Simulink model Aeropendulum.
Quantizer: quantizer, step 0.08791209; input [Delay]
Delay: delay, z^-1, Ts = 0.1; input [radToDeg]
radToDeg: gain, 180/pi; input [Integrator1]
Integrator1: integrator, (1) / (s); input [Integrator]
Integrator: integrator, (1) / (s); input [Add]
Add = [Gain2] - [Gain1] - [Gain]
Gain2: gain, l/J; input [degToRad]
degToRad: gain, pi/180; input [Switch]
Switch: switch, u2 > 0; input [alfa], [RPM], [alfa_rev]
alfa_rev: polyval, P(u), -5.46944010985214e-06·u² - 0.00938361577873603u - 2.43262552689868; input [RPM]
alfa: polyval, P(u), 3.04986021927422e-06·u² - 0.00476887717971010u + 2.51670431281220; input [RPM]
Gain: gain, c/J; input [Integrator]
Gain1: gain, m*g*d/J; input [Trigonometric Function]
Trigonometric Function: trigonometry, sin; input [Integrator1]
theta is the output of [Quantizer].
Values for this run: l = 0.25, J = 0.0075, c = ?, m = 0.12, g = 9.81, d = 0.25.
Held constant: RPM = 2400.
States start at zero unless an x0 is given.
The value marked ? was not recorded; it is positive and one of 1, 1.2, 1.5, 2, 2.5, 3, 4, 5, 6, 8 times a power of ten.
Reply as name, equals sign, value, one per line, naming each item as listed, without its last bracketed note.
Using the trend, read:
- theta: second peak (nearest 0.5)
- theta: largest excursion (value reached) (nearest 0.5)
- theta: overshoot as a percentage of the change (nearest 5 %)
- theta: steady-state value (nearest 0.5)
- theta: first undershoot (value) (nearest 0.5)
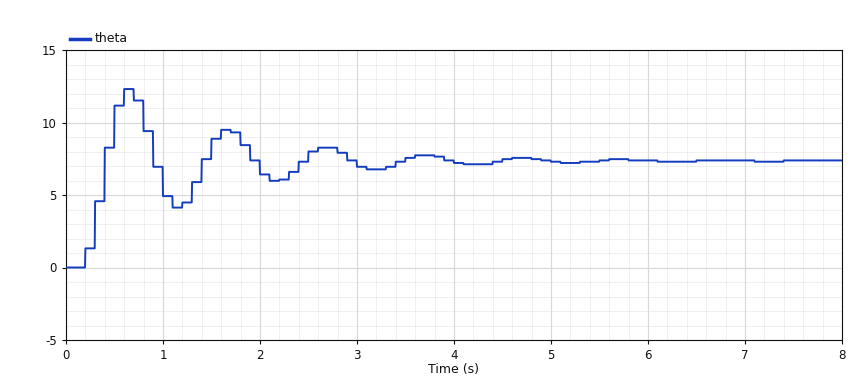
theta: second peak = 9.5
theta: largest excursion (value reached) = 12.5
theta: overshoot as a percentage of the change = 65 %
theta: steady-state value = 7.5
theta: first undershoot (value) = 4.0
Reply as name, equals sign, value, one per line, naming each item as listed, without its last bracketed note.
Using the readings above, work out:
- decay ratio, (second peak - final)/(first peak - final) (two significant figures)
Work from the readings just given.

decay ratio, (second peak - final)/(first peak - final) = 0.40
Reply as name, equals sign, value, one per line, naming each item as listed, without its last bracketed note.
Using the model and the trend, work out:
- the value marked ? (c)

the value marked ? = 0.012
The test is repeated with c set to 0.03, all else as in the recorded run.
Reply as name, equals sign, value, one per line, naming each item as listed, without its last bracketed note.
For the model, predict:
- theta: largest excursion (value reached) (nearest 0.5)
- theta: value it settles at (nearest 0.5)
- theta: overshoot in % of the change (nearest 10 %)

theta: largest excursion (value reached) = 10.0
theta: value it settles at = 7.5
theta: overshoot in % of the change = 30 %
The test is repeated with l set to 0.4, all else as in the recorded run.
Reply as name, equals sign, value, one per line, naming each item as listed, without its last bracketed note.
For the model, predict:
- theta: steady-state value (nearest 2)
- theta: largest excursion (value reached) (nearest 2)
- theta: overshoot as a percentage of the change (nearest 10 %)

theta: steady-state value = 12
theta: largest excursion (value reached) = 20
theta: overshoot as a percentage of the change = 70 %
